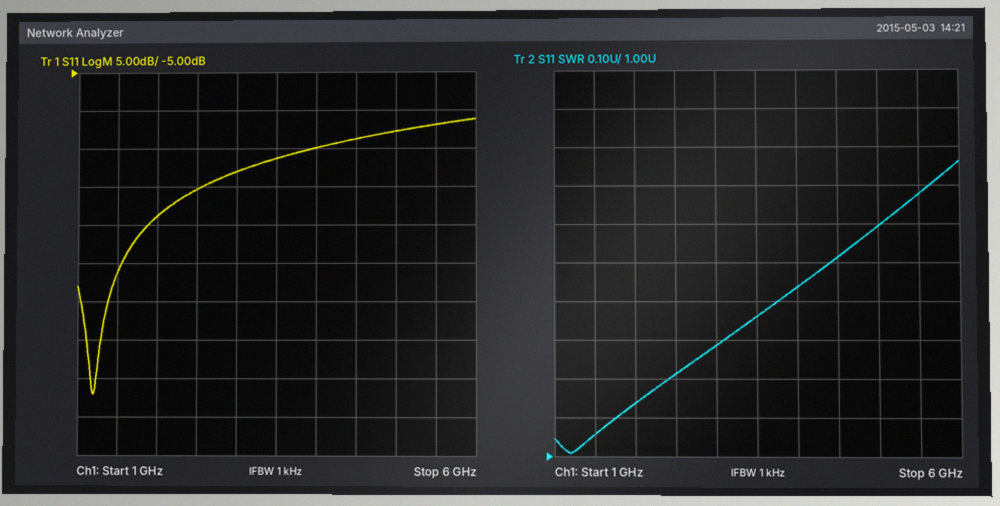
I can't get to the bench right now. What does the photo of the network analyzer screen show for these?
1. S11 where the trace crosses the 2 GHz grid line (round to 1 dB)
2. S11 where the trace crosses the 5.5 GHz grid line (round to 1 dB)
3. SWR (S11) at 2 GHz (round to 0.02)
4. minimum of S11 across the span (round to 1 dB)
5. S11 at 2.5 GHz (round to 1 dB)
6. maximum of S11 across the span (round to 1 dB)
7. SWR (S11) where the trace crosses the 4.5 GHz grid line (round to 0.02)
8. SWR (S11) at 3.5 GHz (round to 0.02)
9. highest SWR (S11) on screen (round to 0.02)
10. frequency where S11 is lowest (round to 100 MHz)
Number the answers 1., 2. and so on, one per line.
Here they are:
1. -24 dB
2. -12 dB
3. 1.14
4. -47 dB
5. -20 dB
6. -11 dB
7. 1.52
8. 1.36
9. 1.76
10. 1.2 GHz
